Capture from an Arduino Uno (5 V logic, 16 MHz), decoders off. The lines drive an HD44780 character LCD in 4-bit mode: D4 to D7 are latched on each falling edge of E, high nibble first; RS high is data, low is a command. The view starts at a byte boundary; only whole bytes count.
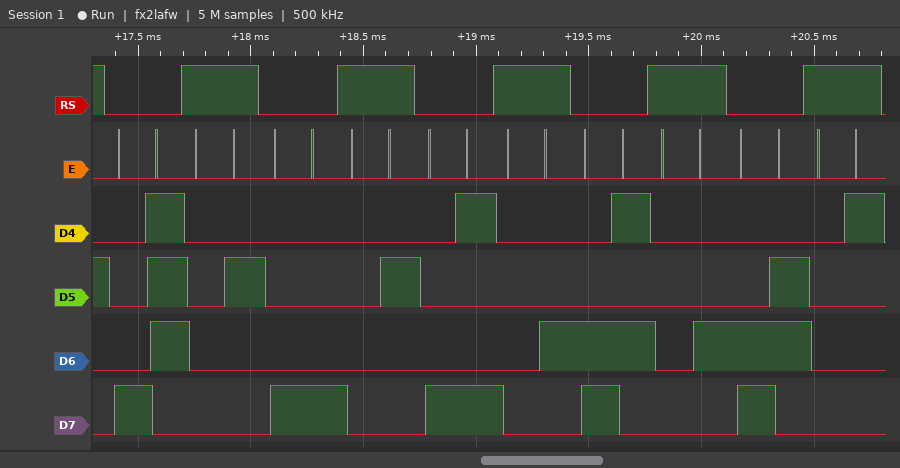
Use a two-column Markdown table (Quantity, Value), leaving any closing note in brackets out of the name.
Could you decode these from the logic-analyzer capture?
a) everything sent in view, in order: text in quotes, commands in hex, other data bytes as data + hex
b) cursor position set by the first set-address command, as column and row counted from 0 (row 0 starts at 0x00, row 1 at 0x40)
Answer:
| Quantity | Value |
|---|---|
| everything sent in view, in order: text in quotes, commands in hex, other data bytes as data + hex | 0x87 data 02 0x88 data 02 0x89 data 04 0xC5 data 04 0xC6 data 01 |
| cursor position set by the first set-address command, as column and row counted from 0 | column 7, row 0 |
